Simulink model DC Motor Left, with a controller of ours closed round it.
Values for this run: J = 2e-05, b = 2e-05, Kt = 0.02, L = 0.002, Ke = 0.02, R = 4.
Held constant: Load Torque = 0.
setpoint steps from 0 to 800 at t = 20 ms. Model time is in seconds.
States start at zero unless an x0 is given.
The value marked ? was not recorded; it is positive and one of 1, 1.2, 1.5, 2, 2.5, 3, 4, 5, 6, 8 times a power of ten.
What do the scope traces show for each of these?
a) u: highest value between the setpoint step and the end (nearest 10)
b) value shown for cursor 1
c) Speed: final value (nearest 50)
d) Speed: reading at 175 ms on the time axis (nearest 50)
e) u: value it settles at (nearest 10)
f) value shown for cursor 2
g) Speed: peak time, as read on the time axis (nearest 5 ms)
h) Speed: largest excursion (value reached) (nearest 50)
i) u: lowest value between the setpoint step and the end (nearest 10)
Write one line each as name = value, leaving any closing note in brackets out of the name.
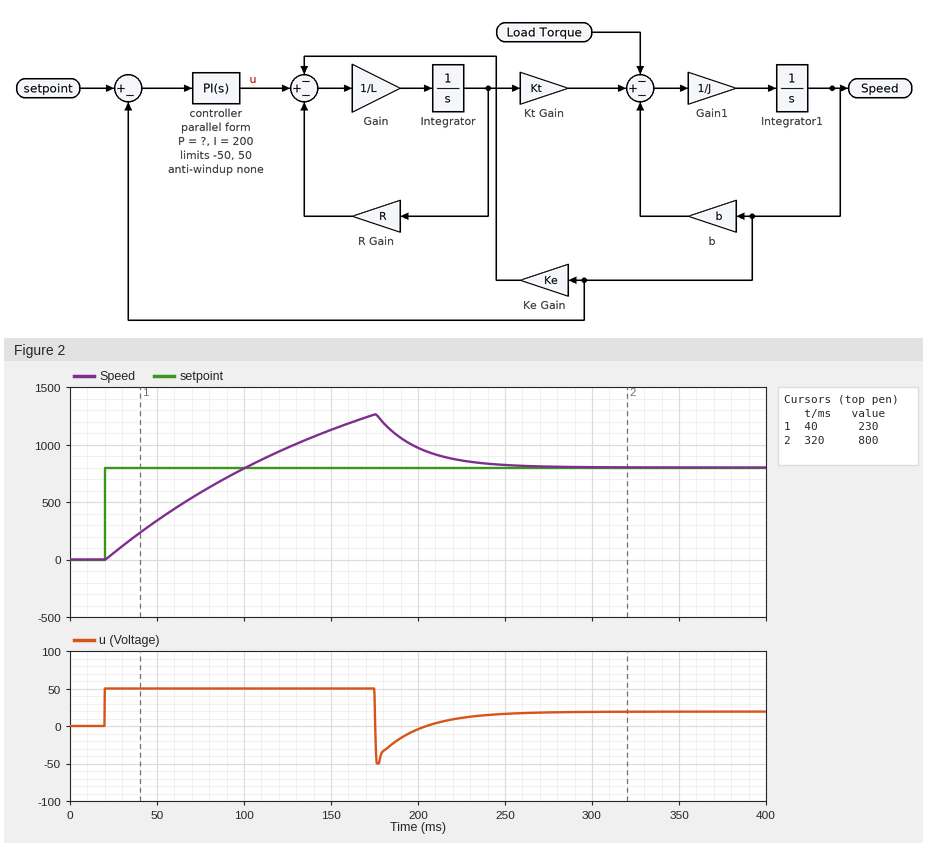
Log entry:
u: highest value between the setpoint step and the end = 50
value shown for cursor 1 = 230
Speed: final value = 800
Speed: reading at 175 ms on the time axis = 1250
u: value it settles at = 20
value shown for cursor 2 = 800
Speed: peak time, as read on the time axis = 175 ms
Speed: largest excursion (value reached) = 1250
u: lowest value between the setpoint step and the end = -50
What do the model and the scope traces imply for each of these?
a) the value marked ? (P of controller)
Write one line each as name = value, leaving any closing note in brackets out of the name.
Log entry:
the value marked ? = 5
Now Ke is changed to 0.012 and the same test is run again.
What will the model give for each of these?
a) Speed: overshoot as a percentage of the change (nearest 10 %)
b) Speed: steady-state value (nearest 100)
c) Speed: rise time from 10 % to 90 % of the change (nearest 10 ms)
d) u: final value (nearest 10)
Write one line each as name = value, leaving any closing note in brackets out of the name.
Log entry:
Speed: overshoot as a percentage of the change = 60 %
Speed: steady-state value = 800
Speed: rise time from 10 % to 90 % of the change = 60 ms
u: final value = 10
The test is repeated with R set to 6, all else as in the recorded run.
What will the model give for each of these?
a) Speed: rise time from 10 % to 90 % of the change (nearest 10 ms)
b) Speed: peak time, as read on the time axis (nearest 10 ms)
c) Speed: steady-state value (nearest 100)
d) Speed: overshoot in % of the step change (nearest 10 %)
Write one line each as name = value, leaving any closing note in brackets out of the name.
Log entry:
Speed: rise time from 10 % to 90 % of the change = 100 ms
Speed: peak time, as read on the time axis = 270 ms
Speed: steady-state value = 800
Speed: overshoot in % of the step change = 60 %
